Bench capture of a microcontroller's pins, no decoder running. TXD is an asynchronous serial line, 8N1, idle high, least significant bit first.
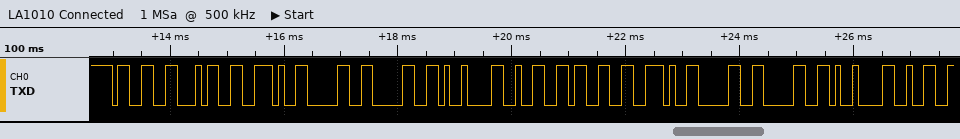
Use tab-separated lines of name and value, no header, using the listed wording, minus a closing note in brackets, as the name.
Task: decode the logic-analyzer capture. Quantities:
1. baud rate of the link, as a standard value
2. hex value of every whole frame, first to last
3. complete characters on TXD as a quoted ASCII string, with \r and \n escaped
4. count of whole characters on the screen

baud rate of the link, as a standard value	9600 baud
hex value of every whole frame, first to last	0x33 0x34 0x2E 0x30 0x30 0x09 0x32 0x33 0x2E 0x30 0x30 0x09 0x32
complete characters on TXD as a quoted ASCII string, with \r and \n escaped	"34.00\t23.00\t2"
count of whole characters on the screen	13
